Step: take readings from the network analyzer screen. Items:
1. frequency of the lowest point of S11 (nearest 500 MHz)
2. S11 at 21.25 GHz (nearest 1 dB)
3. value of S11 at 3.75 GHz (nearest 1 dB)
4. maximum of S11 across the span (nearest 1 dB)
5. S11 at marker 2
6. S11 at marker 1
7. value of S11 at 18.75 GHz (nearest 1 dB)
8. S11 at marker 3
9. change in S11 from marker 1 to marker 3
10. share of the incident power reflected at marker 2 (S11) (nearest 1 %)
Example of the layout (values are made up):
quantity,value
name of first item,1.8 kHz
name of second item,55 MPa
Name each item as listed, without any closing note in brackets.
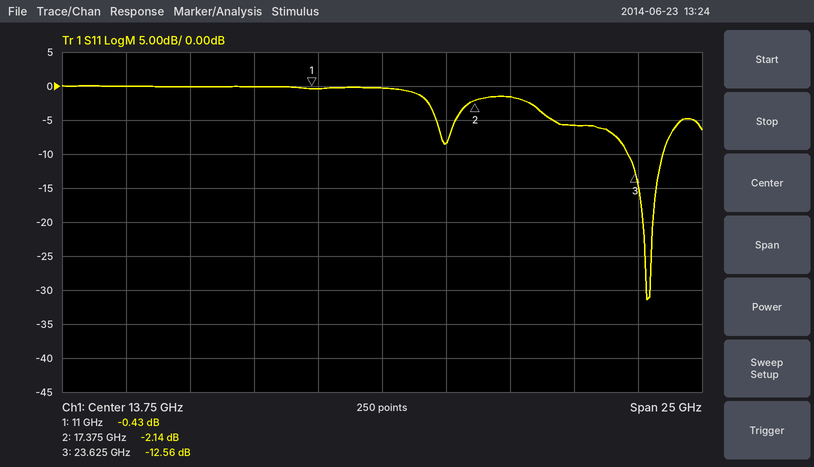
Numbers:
quantity,value
frequency of the lowest point of S11,24.0 GHz
S11 at 21.25 GHz,-6 dB
value of S11 at 3.75 GHz,0 dB
maximum of S11 across the span,0 dB
S11 at marker 2,-2.14 dB
S11 at marker 1,-0.43 dB
value of S11 at 18.75 GHz,-2 dB
S11 at marker 3,-12.56 dB
change in S11 from marker 1 to marker 3,-12.13 dB
share of the incident power reflected at marker 2 (S11),61 %
